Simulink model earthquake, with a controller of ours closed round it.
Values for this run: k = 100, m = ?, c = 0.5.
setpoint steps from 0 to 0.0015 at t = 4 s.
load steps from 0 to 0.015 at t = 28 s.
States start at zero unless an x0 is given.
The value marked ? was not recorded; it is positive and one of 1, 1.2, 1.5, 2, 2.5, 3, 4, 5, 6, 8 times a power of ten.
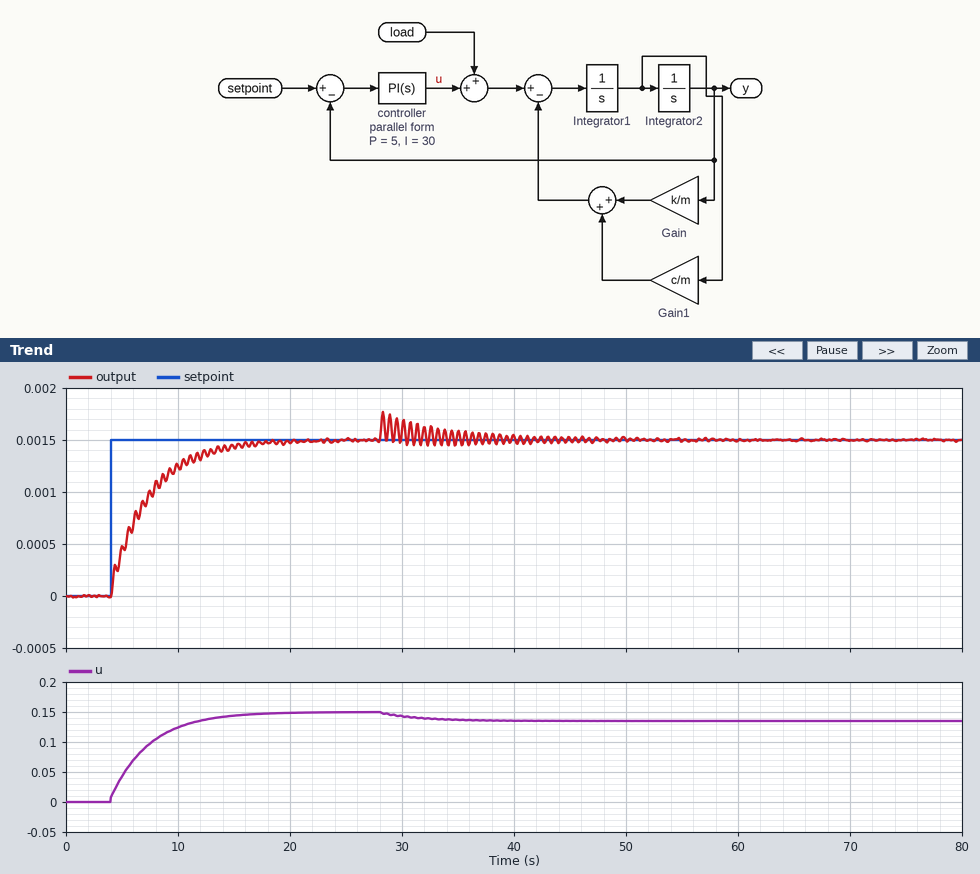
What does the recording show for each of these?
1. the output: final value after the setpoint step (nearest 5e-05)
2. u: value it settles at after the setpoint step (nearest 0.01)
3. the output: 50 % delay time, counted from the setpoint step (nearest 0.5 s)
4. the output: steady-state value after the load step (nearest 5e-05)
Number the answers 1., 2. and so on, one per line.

1. 0.00150
2. 0.15
3. 2.0 s
4. 0.00150
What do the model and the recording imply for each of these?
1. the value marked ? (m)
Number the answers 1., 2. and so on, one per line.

1. 1
